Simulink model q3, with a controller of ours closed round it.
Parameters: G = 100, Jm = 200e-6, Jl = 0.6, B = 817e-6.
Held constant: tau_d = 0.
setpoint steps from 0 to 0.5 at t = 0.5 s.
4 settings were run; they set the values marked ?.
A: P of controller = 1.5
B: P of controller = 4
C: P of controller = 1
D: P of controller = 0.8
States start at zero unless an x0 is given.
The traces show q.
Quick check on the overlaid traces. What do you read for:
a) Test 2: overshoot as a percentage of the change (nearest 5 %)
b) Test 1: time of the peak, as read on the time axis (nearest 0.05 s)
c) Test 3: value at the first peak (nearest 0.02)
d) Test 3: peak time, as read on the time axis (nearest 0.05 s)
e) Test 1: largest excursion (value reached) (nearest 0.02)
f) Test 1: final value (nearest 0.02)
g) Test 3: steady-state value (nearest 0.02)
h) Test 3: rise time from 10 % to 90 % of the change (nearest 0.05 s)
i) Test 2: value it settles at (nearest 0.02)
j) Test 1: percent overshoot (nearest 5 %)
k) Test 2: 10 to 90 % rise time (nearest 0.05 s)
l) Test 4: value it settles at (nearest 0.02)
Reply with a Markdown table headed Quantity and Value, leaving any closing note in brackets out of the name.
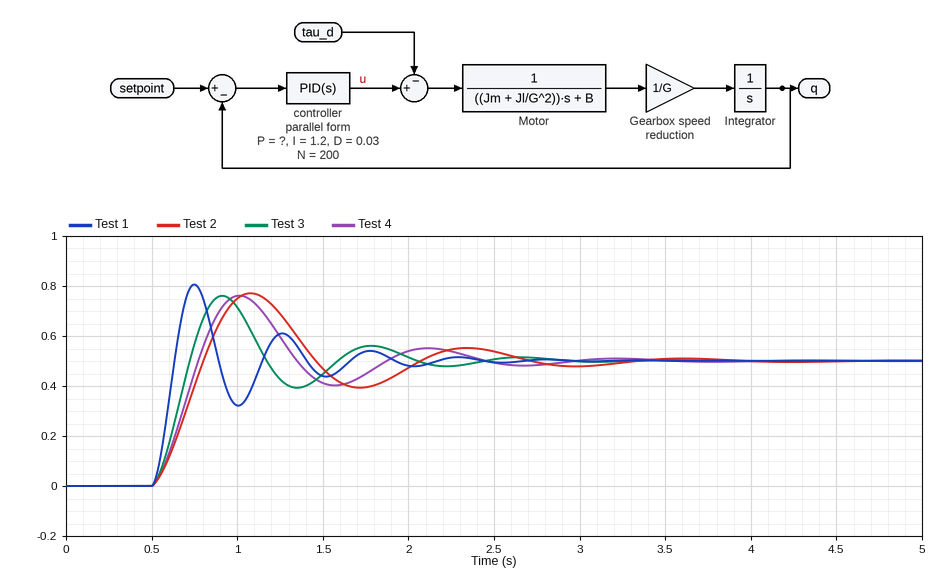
| Quantity | Value |
|---|---|
| Test 2: overshoot as a percentage of the change | 55 % |
| Test 1: time of the peak, as read on the time axis | 0.75 s |
| Test 3: value at the first peak | 0.76 |
| Test 3: peak time, as read on the time axis | 0.90 s |
| Test 1: largest excursion (value reached) | 0.80 |
| Test 1: final value | 0.50 |
| Test 3: steady-state value | 0.50 |
| Test 3: rise time from 10 % to 90 % of the change | 0.15 s |
| Test 2: value it settles at | 0.50 |
| Test 1: percent overshoot | 60 % |
| Test 2: 10 to 90 % rise time | 0.20 s |
| Test 4: value it settles at | 0.50 |
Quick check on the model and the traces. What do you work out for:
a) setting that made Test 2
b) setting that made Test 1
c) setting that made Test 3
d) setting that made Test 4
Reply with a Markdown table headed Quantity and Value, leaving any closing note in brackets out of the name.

| Quantity | Value |
|---|---|
| setting that made Test 2 | D |
| setting that made Test 1 | B |
| setting that made Test 3 | A |
| setting that made Test 4 | C |
